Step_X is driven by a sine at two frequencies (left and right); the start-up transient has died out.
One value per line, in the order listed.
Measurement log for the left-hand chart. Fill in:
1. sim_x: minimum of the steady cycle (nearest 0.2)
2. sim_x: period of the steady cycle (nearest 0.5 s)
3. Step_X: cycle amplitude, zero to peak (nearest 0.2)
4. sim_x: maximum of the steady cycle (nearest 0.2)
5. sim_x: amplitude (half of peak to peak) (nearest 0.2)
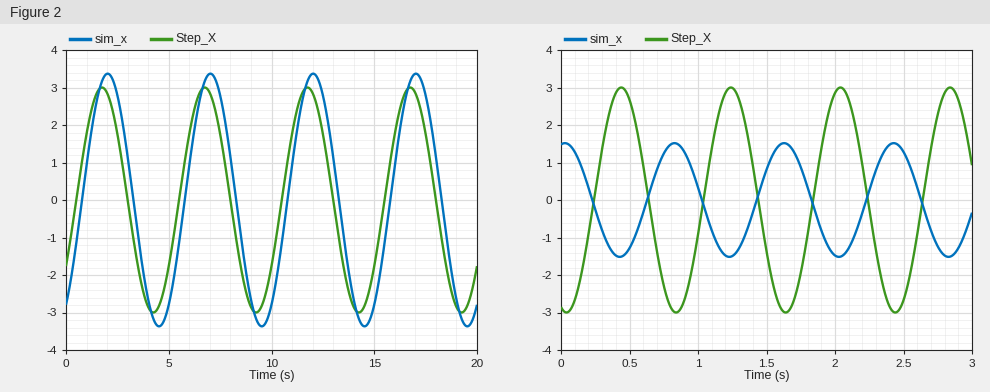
-3.4
5.0 s
3.0
3.4
3.4
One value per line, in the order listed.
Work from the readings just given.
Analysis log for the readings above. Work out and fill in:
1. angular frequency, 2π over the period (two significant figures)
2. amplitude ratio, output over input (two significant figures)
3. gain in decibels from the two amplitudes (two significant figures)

1.3 rad/s
1.1
1.1 dB
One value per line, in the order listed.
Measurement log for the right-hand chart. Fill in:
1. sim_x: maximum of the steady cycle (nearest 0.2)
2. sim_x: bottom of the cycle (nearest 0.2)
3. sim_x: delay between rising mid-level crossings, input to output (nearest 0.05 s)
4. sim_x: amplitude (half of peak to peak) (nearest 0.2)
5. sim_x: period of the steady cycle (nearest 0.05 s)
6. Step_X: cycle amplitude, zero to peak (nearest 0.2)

1.6
-1.6
0.40 s
1.6
0.80 s
3.0
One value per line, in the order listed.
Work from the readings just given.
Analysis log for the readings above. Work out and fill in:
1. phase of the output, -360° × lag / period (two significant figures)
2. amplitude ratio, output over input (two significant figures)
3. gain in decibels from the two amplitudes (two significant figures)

-180°
0.53
-5.5 dB
